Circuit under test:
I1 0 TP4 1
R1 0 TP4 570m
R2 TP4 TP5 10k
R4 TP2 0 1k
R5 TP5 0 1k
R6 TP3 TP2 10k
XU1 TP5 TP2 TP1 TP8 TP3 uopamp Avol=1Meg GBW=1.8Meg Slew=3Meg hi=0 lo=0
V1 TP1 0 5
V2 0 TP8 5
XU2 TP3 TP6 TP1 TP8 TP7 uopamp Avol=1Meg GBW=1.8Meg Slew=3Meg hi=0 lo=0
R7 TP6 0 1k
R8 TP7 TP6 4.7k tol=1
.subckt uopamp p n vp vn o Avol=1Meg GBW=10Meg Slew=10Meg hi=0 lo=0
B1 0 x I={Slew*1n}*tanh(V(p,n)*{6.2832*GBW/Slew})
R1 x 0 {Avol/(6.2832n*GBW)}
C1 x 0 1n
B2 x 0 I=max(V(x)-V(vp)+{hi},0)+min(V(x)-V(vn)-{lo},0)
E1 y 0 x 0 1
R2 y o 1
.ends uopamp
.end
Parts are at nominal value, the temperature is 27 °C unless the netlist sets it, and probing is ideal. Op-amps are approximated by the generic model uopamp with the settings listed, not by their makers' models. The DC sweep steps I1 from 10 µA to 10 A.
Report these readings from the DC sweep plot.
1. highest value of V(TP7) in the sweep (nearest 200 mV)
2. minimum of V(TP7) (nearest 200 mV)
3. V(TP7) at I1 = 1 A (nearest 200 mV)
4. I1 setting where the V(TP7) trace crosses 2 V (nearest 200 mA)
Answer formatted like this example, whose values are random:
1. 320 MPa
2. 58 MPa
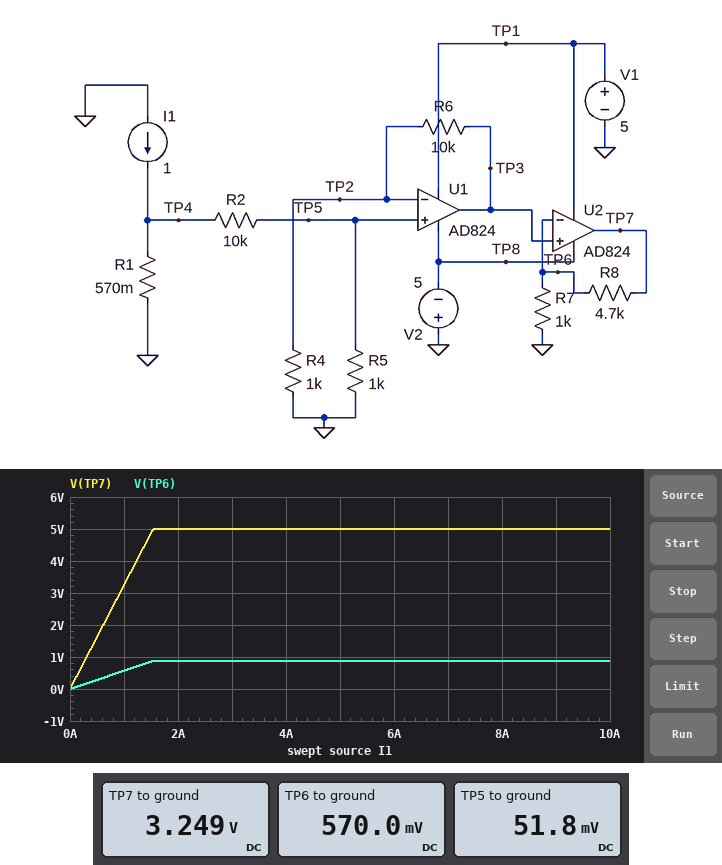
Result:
1. 5.0 V
2. 0 V
3. 3.2 V
4. 600 mA
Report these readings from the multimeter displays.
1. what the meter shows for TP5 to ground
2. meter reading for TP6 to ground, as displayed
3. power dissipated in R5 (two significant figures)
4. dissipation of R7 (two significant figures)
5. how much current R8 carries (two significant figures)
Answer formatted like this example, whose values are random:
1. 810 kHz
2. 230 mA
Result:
1. 51.8 mV
2. 570.0 mV
3. 2.7 µW
4. 320 µW
5. 570 µA
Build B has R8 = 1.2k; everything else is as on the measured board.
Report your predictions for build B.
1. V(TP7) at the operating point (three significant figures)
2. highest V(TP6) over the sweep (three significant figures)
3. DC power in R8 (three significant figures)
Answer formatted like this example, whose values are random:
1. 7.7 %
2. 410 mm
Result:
1. 1.25 V
2. 2.27 V
3. 390 µW
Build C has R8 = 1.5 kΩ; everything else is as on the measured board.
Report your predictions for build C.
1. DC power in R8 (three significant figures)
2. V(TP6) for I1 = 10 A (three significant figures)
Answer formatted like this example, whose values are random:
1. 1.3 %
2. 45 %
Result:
1. 487 µW
2. 2.00 V
